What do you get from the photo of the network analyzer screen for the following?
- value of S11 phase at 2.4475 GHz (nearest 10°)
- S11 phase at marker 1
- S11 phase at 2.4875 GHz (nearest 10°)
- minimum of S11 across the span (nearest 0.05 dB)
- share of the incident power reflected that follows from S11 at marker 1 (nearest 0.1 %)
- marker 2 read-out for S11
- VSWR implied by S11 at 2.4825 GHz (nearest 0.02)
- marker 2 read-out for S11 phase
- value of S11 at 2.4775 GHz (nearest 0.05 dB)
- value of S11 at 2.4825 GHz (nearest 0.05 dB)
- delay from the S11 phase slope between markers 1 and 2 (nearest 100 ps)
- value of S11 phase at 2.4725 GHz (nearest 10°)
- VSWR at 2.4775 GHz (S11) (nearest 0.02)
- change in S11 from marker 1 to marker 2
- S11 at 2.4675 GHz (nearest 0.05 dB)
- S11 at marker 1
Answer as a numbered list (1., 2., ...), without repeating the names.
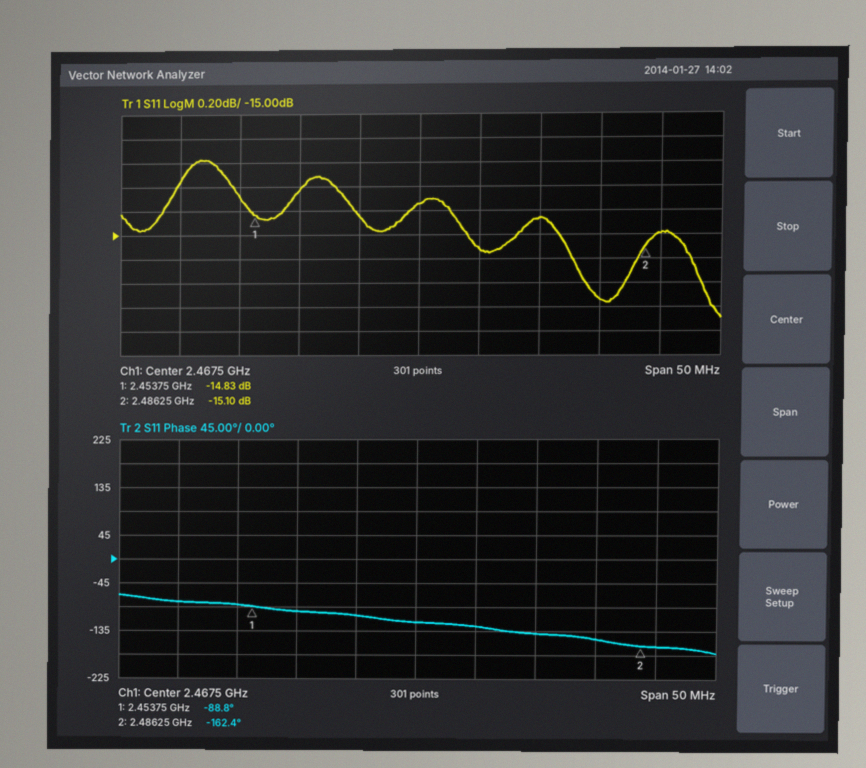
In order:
1. -80°
2. -88.8°
3. -160°
4. -15.70 dB
5. 3.3 %
6. -15.10 dB
7. 1.40
8. -162.4°
9. -14.85 dB
10. -15.55 dB
11. 6.3 ns
12. -130°
13. 1.44
14. -0.27 dB
15. -14.75 dB
16. -14.83 dB
